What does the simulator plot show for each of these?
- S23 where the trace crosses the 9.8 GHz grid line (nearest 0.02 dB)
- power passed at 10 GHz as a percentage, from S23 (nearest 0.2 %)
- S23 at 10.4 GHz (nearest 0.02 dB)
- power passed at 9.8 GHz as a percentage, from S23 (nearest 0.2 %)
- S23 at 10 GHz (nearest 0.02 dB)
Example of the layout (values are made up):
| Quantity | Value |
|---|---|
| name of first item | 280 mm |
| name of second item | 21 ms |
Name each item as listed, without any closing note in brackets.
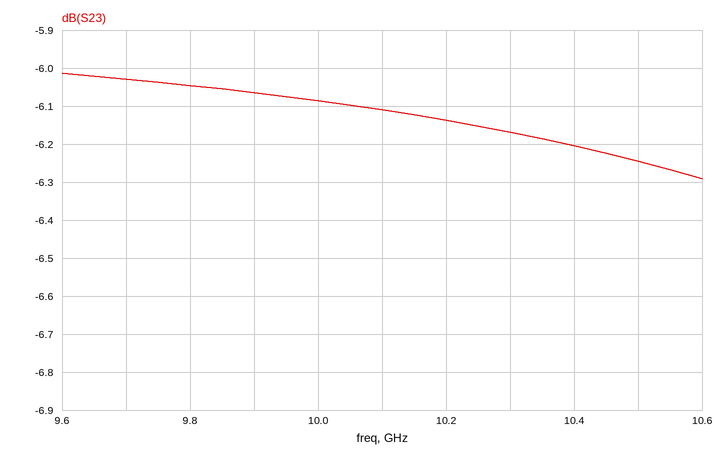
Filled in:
| Quantity | Value |
|---|---|
| S23 where the trace crosses the 9.8 GHz grid line | -6.04 dB |
| power passed at 10 GHz as a percentage, from S23 | 24.6 % |
| S23 at 10.4 GHz | -6.20 dB |
| power passed at 9.8 GHz as a percentage, from S23 | 24.8 % |
| S23 at 10 GHz | -6.08 dB |
